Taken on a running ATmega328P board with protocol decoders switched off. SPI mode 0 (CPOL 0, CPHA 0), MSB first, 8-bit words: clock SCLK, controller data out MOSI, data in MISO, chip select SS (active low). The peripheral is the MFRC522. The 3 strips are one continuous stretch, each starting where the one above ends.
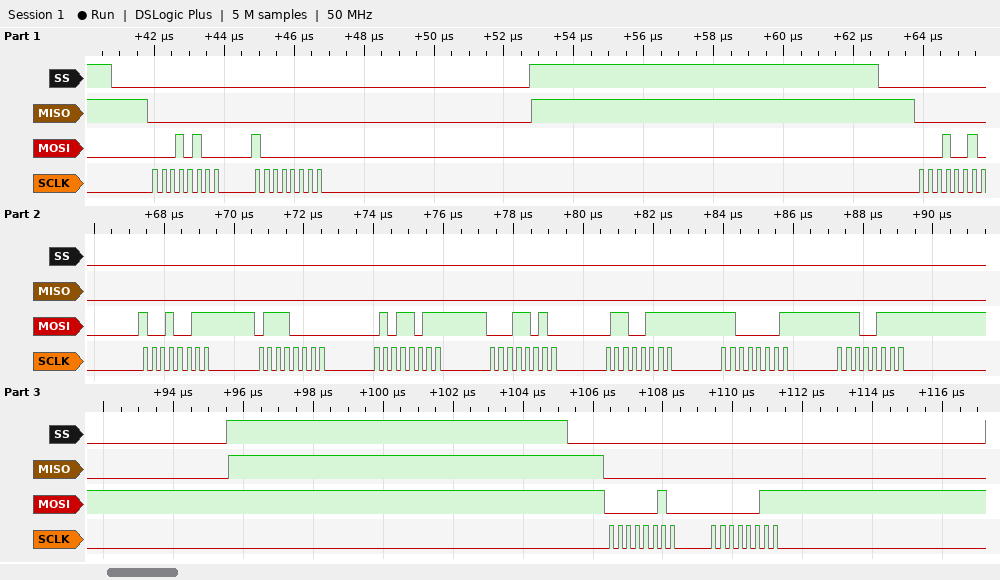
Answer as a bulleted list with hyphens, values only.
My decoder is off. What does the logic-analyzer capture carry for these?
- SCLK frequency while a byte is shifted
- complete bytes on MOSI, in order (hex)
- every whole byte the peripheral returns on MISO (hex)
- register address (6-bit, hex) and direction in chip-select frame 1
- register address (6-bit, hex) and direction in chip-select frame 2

- 4 MHz
- 14 80 12 93 70 5B 1A 67 C1 E7 02 03
- 00 00 00 00 00 00 00 00 00 00 00 00
- 0x0A write
- 0x09 write
